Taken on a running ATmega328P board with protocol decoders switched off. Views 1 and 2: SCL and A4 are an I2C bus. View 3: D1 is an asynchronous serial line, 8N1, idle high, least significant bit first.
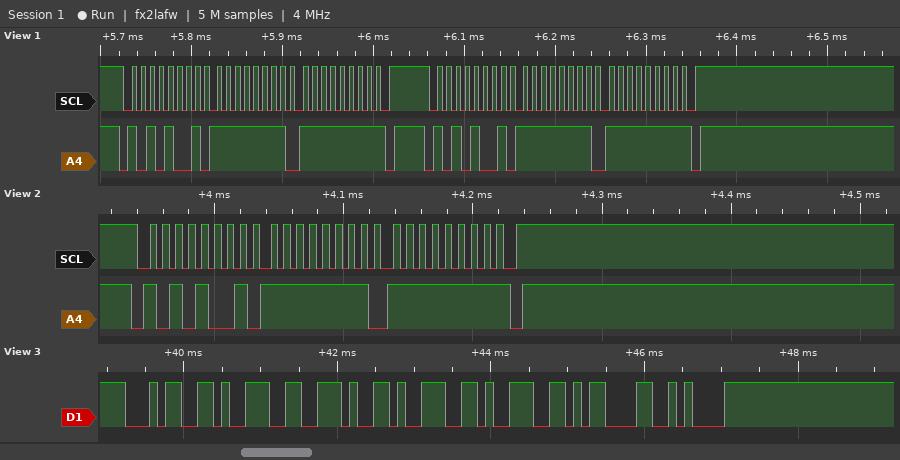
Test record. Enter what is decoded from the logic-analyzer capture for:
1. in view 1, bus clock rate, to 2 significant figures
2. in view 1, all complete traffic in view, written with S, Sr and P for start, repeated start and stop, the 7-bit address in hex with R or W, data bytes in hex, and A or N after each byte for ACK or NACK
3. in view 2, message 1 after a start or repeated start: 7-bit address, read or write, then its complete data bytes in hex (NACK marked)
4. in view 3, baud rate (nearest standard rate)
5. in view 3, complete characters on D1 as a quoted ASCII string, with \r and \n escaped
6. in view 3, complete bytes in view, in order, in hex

100 kHz
S 54R A FF A FF N P S 54R A FF A FF N P
0x54 read: FF FF NACK
9600 baud
"49.99\r\n"
34 39 2E 39 39 0D 0A
